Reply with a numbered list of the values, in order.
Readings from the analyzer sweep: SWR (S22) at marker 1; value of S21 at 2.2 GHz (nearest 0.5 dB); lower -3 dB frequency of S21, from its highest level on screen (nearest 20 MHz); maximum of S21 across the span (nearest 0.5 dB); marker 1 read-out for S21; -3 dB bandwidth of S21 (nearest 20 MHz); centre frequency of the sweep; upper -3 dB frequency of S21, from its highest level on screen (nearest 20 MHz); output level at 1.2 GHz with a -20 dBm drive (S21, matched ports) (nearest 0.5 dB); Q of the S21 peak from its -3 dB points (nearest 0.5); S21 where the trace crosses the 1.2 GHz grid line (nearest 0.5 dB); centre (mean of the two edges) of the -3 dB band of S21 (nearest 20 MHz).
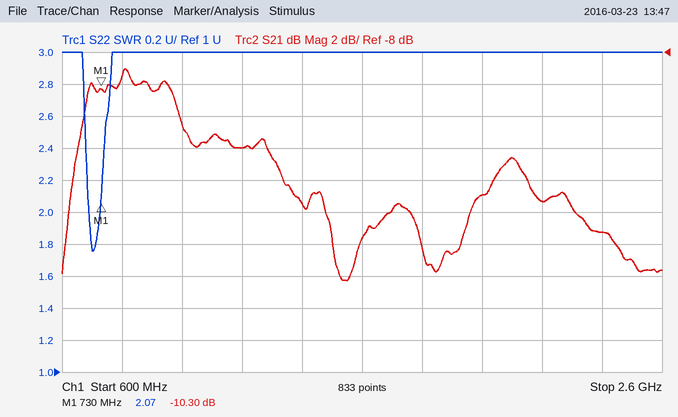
1. 2.07
2. -17.5 dB
3. 680 MHz
4. -9.0 dB
5. -10.30 dB
6. 320 MHz
7. 1.6 GHz
8. 1.00 GHz
9. -34.0 dBm
10. 2.5
11. -14.0 dB
12. 840 MHz
